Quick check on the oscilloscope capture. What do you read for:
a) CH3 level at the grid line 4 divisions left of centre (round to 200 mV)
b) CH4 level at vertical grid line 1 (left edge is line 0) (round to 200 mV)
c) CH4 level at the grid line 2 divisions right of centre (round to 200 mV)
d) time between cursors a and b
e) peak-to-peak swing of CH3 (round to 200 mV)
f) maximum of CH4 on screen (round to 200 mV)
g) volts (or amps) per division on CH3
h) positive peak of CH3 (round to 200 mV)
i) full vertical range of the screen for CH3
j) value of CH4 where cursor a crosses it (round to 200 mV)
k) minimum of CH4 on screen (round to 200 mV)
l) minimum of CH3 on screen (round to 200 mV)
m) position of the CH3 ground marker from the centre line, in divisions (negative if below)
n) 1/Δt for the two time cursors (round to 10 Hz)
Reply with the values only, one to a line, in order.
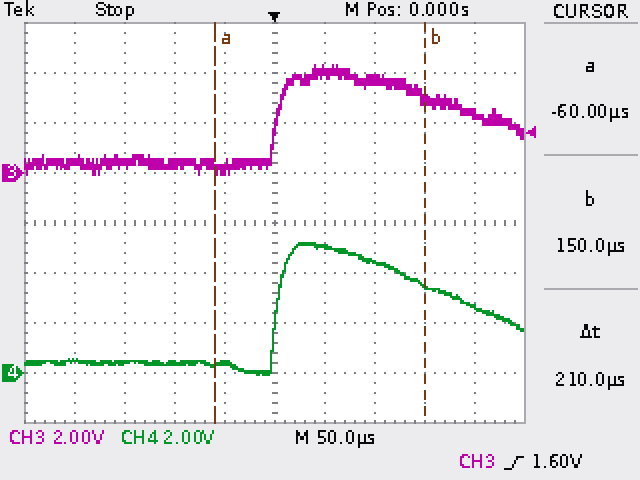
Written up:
400 mV
400 mV
4.4 V
210 µs
4.4 V
5.2 V
2 V
4.4 V
16 V
400 mV
0.0 V
0.0 V
+1.0 div
4.76 kHz
